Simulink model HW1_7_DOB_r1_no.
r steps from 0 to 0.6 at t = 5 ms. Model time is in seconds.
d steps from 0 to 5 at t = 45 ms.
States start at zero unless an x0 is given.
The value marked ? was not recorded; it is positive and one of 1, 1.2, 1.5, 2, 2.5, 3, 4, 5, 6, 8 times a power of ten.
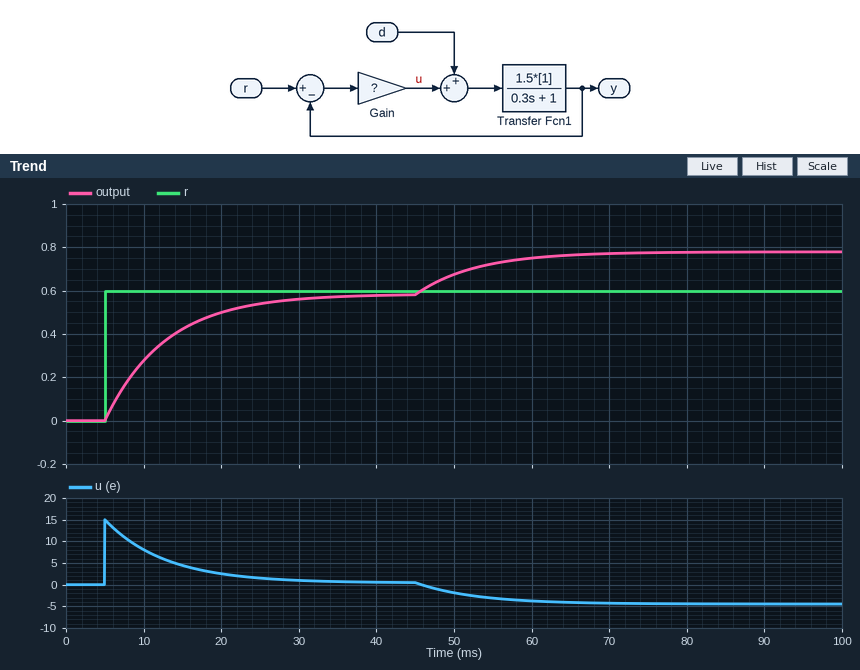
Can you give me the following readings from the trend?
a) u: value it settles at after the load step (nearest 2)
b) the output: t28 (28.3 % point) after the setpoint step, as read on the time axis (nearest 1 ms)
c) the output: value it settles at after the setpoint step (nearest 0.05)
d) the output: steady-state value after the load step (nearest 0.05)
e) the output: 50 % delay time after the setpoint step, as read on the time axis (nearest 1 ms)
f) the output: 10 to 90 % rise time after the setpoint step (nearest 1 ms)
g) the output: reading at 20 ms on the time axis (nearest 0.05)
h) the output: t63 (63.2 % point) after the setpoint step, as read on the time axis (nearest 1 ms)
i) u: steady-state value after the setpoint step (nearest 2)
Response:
-4
8 ms
0.60
0.80
10 ms
17 ms
0.50
13 ms
0
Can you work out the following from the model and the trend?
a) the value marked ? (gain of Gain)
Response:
25
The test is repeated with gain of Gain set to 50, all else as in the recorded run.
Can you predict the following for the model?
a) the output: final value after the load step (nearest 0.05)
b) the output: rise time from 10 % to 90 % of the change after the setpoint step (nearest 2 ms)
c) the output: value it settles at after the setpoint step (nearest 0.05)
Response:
0.70
8 ms
0.60
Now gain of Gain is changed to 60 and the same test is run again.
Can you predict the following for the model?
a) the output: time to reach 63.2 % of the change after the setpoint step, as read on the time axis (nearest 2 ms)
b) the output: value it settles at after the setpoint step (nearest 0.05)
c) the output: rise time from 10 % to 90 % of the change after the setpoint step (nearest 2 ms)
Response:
8 ms
0.60
8 ms
